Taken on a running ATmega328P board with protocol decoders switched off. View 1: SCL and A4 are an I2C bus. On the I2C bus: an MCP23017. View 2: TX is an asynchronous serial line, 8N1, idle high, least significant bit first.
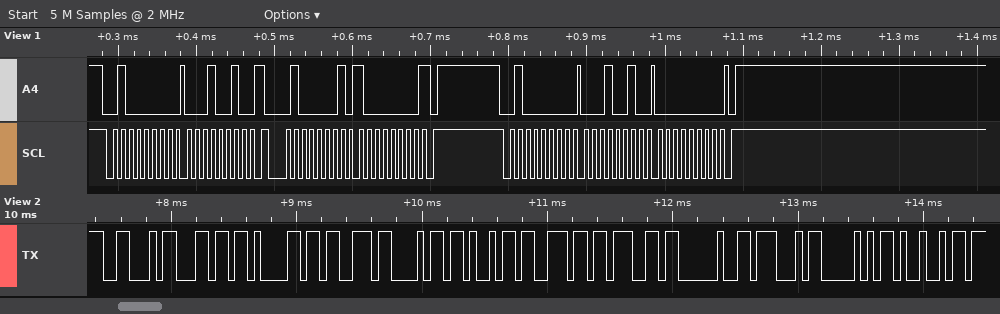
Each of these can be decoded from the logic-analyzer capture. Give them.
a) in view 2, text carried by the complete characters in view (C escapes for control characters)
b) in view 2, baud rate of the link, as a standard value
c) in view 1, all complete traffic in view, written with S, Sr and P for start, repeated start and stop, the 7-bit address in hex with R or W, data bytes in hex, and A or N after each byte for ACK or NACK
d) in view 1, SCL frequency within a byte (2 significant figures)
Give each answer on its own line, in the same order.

"Flashing GPI"
19200 baud
S 20W A 12 A Sr 20R A 80 N P S 20W A 12 A 00 A P
100 kHz
